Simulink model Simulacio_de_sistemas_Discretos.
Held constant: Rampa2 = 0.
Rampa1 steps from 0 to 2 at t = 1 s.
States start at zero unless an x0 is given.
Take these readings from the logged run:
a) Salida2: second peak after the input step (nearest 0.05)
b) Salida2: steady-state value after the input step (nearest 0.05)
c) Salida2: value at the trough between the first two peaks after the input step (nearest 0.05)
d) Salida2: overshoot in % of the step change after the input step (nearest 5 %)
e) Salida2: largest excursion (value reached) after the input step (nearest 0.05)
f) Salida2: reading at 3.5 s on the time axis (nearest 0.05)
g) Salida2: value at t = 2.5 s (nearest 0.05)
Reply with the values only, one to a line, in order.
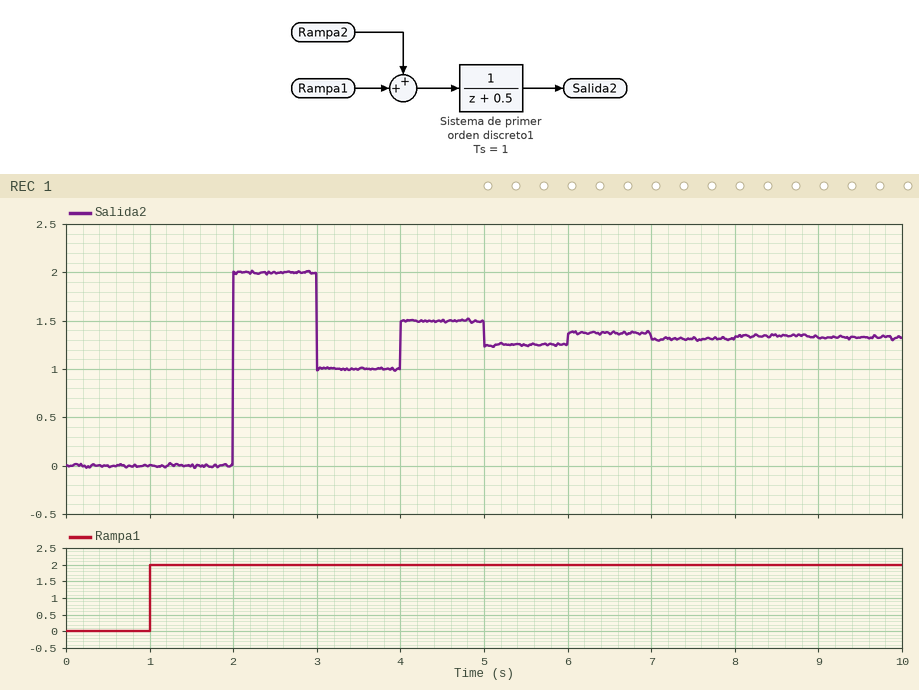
1.50
1.35
1.00
50 %
2.00
1.00
2.00
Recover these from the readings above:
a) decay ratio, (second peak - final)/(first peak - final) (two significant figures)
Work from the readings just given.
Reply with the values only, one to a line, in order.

0.23
